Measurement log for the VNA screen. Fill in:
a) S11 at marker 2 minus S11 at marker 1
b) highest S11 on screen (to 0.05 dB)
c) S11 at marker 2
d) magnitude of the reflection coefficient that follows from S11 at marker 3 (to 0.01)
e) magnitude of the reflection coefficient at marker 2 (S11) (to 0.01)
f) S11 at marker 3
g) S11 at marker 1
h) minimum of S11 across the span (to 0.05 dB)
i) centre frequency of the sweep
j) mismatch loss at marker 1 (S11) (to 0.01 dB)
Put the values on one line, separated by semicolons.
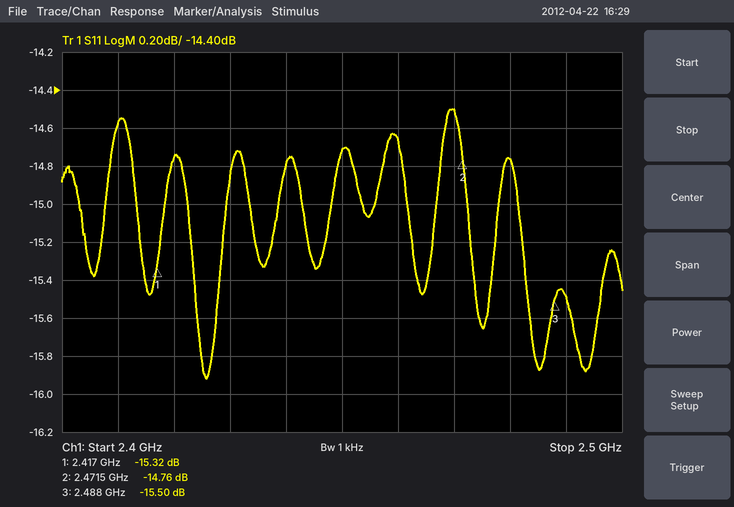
0.56 dB; -14.50 dB; -14.76 dB; 0.17; 0.18; -15.50 dB; -15.32 dB; -15.90 dB; 2.45 GHz; 0.13 dB
